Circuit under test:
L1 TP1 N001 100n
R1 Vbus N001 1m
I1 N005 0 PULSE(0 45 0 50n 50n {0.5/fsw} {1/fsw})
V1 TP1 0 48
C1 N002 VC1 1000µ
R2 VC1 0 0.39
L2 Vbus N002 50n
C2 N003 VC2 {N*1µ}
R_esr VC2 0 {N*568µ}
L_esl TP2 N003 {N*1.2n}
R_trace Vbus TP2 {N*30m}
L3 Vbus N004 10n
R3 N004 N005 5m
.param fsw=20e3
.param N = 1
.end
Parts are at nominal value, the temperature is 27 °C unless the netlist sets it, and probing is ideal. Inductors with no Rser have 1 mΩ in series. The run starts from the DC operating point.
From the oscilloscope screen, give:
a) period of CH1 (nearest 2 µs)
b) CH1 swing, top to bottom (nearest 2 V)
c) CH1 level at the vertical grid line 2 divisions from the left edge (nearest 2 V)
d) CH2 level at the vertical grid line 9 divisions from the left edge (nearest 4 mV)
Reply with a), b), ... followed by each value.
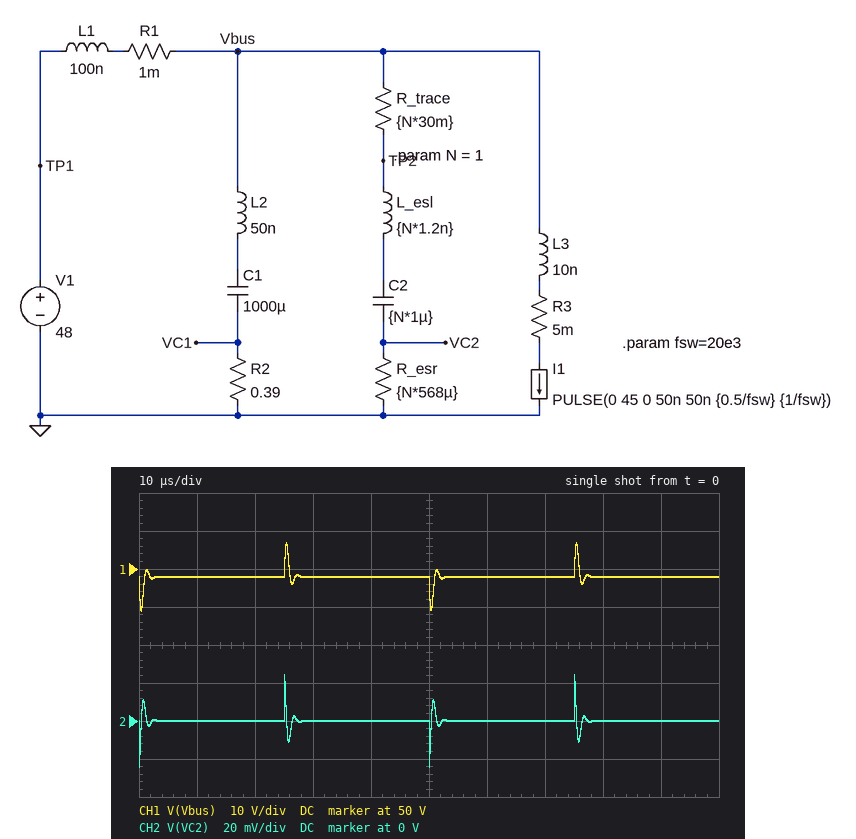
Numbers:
a) 50 µs
b) 18 V
c) 48 V
d) 0 V
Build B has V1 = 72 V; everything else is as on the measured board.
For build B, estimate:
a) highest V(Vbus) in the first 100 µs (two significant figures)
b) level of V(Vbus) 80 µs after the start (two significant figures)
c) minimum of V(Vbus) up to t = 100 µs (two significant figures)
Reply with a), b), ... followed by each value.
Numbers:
a) 81 V
b) 72 V
c) 63 V
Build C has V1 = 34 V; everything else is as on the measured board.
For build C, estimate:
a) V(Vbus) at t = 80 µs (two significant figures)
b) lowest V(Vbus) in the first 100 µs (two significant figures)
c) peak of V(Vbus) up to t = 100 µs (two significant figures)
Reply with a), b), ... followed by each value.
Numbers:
a) 34 V
b) 25 V
c) 43 V
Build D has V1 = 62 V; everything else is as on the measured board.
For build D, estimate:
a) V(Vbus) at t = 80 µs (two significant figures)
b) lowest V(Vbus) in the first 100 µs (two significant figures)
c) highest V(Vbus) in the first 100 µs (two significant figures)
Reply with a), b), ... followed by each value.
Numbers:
a) 62 V
b) 53 V
c) 71 V
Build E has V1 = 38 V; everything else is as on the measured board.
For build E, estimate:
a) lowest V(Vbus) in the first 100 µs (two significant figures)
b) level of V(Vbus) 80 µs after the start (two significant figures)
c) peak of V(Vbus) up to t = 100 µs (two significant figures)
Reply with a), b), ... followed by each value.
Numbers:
a) 29 V
b) 38 V
c) 47 V
